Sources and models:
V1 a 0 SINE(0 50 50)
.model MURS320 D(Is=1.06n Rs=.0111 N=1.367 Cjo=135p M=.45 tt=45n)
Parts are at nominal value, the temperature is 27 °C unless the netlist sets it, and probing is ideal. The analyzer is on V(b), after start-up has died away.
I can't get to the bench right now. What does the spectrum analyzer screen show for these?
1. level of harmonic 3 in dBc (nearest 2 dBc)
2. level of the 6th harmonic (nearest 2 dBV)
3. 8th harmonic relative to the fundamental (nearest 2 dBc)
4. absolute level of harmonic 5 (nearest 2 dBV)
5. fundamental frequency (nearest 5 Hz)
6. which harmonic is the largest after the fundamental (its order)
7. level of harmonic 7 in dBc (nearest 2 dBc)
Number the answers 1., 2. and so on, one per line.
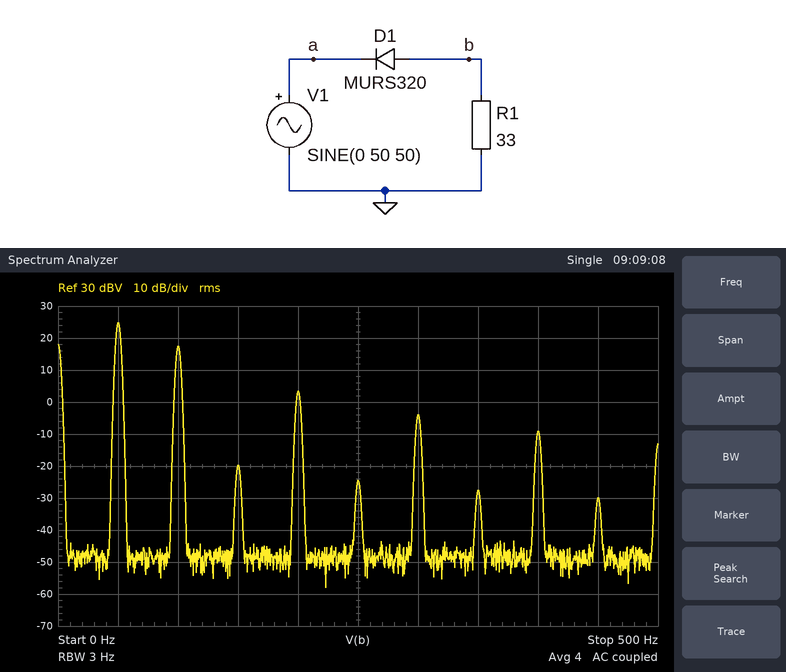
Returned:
1. -44 dBc
2. -4 dBV
3. -34 dBc
4. -24 dBV
5. 50 Hz
6. 2
7. -52 dBc
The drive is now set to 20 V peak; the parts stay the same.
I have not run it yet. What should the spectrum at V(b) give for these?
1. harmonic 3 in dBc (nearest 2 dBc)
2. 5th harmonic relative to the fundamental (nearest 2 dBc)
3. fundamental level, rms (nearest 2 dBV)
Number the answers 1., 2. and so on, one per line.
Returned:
1. -36 dBc
2. -42 dBc
3. 16 dBV
